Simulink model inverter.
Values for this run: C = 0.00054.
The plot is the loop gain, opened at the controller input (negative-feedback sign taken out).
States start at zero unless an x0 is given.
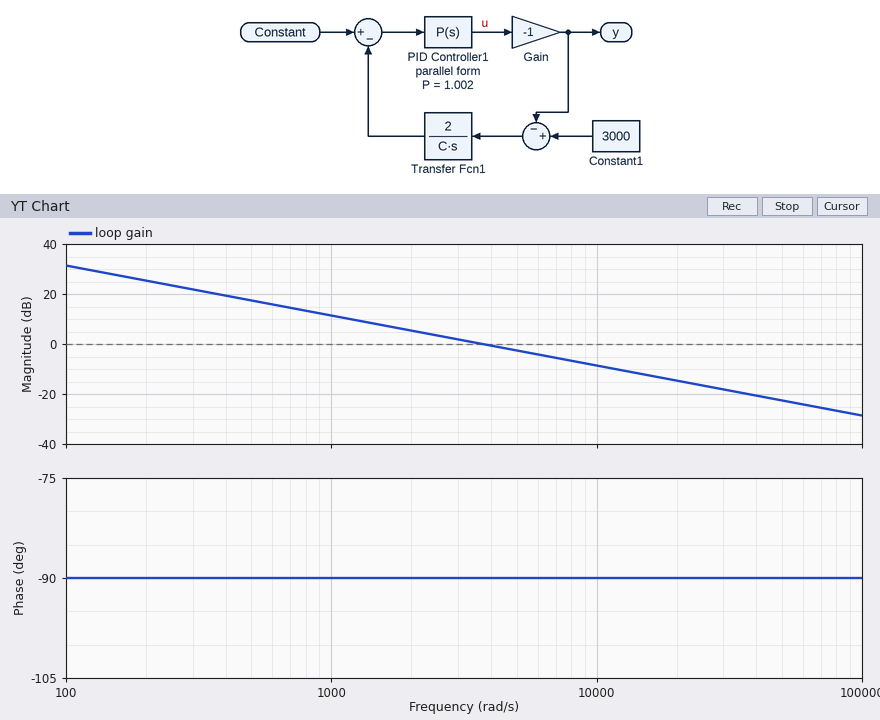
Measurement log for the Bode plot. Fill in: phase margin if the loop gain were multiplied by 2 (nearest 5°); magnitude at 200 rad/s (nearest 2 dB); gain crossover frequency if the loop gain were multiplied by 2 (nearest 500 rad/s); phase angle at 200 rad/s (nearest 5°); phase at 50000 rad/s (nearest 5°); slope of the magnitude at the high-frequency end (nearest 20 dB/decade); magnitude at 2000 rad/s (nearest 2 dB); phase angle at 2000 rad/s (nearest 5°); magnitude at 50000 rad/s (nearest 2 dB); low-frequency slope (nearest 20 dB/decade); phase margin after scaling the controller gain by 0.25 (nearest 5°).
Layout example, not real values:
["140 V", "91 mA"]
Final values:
["90°", "26 dB", "7500 rad/s", "-90°", "-90°", "-20 dB/decade", "6 dB", "-90°", "-22 dB", "-20 dB/decade", "90°"]
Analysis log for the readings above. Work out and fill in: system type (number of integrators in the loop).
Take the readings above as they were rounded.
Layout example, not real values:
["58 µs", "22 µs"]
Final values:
["1"]
